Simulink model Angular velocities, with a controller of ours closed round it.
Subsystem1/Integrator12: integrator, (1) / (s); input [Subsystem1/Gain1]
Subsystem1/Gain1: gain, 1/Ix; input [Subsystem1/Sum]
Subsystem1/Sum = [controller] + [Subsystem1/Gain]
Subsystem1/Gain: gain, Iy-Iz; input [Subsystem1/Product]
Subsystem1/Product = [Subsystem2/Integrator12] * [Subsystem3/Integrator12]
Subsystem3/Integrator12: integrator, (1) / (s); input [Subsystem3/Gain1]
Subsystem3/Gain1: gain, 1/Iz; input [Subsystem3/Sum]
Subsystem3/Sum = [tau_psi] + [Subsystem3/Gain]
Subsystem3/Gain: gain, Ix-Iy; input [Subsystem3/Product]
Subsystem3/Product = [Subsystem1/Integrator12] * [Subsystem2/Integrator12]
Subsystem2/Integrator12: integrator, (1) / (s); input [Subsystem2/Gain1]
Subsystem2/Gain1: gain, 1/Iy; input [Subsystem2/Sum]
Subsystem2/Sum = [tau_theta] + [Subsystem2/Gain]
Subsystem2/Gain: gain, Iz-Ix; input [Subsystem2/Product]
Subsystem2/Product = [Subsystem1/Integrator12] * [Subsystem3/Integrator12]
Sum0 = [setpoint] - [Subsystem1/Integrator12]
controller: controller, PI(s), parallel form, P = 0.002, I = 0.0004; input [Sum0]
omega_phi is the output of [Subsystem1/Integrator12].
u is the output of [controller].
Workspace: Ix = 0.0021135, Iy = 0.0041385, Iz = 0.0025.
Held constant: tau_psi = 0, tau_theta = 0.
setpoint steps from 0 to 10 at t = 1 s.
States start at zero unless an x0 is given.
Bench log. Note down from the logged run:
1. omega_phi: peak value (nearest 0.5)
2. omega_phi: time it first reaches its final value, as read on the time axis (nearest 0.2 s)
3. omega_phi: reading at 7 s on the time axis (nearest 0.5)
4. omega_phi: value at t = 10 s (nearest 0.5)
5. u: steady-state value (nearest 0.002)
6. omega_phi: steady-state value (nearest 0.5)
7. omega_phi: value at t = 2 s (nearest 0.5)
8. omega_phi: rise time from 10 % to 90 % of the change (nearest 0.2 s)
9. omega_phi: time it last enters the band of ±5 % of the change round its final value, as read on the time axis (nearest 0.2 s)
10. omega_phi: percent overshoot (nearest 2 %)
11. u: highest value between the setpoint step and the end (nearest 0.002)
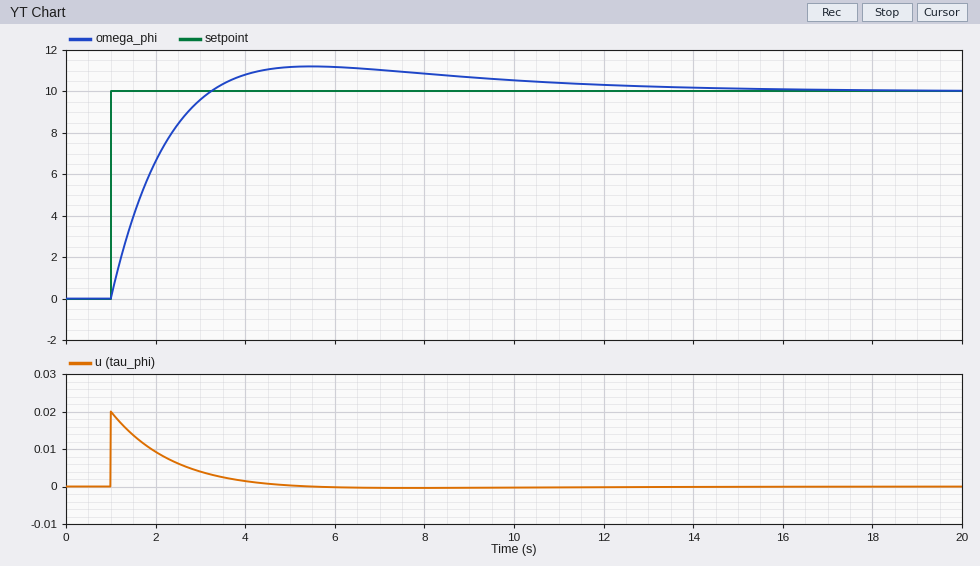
11.0
3.2 s
11.0
10.5
0.000
10.0
6.5
1.6 s
10.2 s
12 %
0.020
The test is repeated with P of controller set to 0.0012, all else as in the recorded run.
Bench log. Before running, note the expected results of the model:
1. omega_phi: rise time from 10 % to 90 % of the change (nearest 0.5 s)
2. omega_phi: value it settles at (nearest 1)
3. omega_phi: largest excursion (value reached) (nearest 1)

2.0 s
10
12
